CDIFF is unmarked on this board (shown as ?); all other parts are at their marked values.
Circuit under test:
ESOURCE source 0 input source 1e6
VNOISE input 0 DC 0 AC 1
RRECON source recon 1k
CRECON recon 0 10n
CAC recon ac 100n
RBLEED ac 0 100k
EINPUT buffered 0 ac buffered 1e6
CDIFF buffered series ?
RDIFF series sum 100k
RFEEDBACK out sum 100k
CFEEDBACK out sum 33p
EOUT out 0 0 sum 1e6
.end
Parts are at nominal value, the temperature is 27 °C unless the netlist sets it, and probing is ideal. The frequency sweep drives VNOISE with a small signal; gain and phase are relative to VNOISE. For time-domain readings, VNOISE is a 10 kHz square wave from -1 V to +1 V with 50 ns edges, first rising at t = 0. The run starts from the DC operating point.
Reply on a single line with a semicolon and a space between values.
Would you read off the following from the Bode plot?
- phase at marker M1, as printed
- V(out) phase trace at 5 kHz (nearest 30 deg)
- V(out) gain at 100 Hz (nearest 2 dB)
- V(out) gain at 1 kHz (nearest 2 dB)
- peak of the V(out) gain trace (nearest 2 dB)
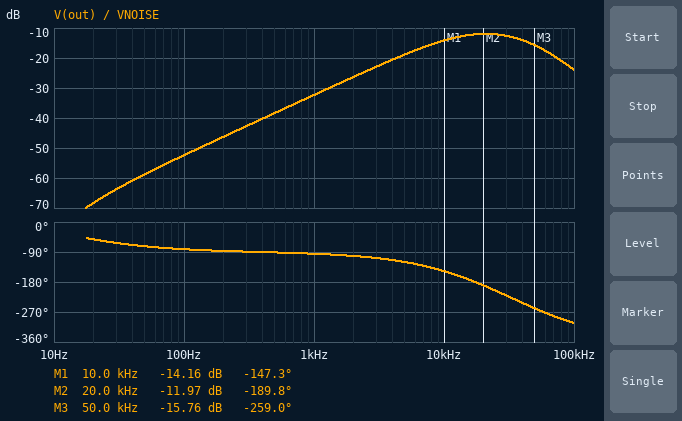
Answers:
-147.3 deg; -120 deg; -52 dB; -32 dB; -12 dB
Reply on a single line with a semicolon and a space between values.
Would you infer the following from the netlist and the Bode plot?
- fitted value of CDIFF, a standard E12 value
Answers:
39 pF
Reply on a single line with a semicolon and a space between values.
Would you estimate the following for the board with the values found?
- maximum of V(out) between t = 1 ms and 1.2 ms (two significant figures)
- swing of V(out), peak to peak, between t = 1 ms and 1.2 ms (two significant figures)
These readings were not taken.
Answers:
370 mV; 730 mV
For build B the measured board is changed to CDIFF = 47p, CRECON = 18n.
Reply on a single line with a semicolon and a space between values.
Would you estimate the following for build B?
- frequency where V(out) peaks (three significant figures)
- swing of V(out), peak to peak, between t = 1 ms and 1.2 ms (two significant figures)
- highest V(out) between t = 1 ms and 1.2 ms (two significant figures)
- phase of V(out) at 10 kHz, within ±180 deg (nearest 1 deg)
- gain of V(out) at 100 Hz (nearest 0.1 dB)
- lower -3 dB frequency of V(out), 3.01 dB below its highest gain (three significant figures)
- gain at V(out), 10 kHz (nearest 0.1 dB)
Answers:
15.2 kHz; 550 mV; 280 mV; -166 deg; -50.8 dB; 5.76 kHz; -14.8 dB
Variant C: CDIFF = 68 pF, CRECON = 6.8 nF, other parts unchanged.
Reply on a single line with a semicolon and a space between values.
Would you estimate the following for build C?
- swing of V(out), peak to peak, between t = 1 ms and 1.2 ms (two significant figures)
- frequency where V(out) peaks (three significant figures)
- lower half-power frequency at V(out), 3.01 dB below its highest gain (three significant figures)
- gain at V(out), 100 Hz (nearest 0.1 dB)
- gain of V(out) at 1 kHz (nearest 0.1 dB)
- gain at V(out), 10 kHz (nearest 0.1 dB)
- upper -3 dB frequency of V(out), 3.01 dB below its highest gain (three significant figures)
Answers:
1.3 V; 20.2 kHz; 8.78 kHz; -47.6 dB; -27.5 dB; -9.1 dB; 41.9 kHz
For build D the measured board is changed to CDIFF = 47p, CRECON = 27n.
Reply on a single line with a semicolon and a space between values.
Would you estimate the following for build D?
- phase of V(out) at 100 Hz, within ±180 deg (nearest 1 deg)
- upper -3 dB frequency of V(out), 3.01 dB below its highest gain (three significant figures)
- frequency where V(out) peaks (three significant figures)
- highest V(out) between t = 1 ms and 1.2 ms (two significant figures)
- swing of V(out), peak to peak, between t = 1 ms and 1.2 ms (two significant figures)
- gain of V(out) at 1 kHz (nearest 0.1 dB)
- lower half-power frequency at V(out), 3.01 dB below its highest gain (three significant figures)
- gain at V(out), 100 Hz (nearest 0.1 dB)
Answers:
-82 deg; 33.1 kHz; 12.5 kHz; 190 mV; 380 mV; -30.8 dB; 4.31 kHz; -50.8 dB
